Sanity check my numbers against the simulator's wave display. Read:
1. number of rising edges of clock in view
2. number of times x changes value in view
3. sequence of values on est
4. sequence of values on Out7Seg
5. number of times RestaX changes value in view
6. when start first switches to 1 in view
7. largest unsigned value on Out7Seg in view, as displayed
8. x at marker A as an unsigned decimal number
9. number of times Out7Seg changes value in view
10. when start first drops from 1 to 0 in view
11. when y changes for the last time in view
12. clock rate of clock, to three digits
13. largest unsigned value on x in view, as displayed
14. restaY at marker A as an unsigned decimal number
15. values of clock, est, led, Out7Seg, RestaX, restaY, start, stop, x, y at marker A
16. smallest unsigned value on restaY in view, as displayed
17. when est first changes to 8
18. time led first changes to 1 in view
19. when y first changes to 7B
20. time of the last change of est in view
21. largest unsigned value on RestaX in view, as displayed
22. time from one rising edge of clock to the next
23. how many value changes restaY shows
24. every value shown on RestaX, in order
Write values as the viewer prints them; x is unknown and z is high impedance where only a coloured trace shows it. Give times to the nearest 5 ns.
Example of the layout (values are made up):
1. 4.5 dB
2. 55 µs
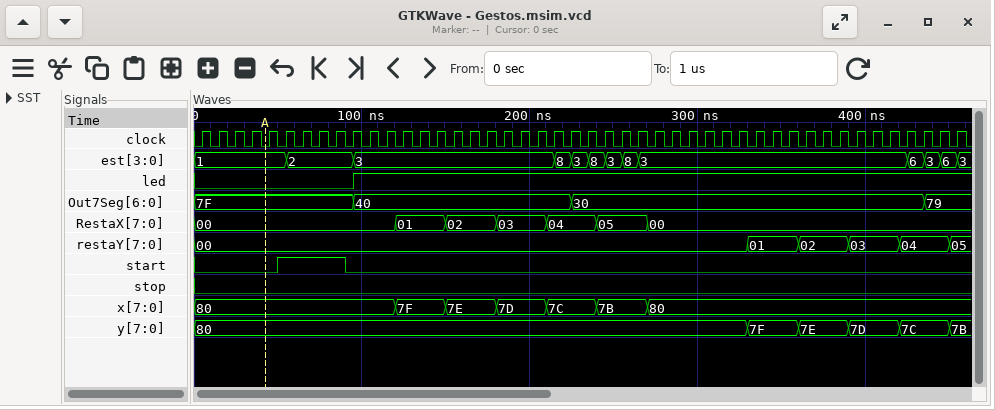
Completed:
1. 46
2. 6
3. 1, 2, 3, 8, 3, 8, 3, 8, 3, 6, 3, 6, 3
4. 7F, 40, 30, 79
5. 6
6. 50 ns
7. 7F
8. 128
9. 3
10. 90 ns
11. 450 ns
12. 100 MHz
13. 80
14. 0
15. clock=0, est=1, led=0, Out7Seg=7F, RestaX=00, restaY=00, start=0, stop=0, x=80, y=80
16. 00
17. 215 ns
18. 95 ns
19. 450 ns
20. 455 ns
21. 05
22. 10 ns
23. 5
24. 00, 01, 02, 03, 04, 05, 00
